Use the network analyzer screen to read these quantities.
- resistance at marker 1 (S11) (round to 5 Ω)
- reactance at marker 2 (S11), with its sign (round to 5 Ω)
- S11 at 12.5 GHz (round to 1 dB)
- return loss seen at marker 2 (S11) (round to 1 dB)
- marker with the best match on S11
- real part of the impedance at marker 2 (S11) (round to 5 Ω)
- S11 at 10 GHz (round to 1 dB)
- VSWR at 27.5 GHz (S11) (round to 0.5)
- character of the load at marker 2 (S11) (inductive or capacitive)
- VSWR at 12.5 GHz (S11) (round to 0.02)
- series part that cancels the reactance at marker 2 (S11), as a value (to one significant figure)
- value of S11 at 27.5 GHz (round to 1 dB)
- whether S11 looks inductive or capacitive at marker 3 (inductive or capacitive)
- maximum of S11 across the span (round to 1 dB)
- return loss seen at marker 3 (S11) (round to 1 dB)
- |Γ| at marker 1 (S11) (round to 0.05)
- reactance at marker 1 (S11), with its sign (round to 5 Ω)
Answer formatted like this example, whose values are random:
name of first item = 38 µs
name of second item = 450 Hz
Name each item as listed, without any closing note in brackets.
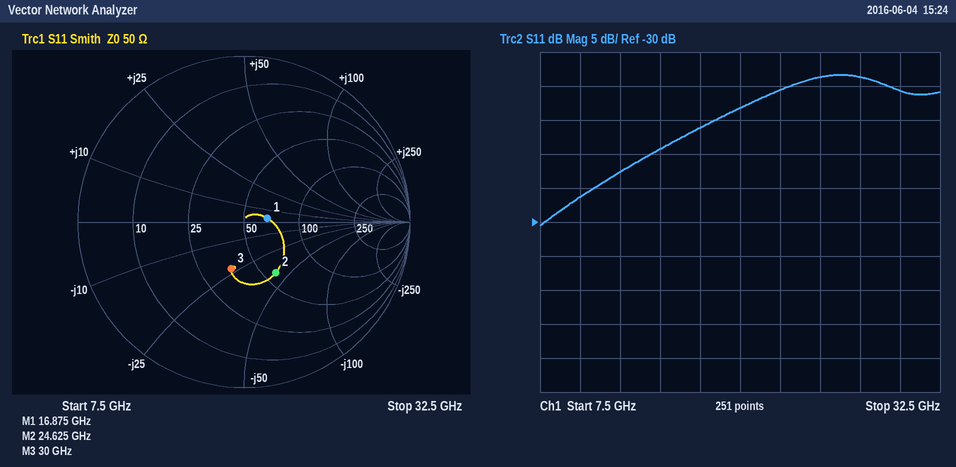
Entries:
resistance at marker 1 (S11) = 65 Ω
reactance at marker 2 (S11), with its sign = -40 Ω
S11 at 12.5 GHz = -23 dB
return loss seen at marker 2 (S11) = 9 dB
marker with the best match on S11 = marker 1
real part of the impedance at marker 2 (S11) = 60 Ω
S11 at 10 GHz = -26 dB
VSWR at 27.5 GHz (S11) = 2.0
character of the load at marker 2 (S11) = capacitive
VSWR at 12.5 GHz (S11) = 1.16
series part that cancels the reactance at marker 2 (S11), as a value = 300 pH
value of S11 at 27.5 GHz = -9 dB
whether S11 looks inductive or capacitive at marker 3 = capacitive
maximum of S11 across the span = -8 dB
return loss seen at marker 3 (S11) = 11 dB
|Γ| at marker 1 (S11) = 0.15
reactance at marker 1 (S11), with its sign = +5 Ω
